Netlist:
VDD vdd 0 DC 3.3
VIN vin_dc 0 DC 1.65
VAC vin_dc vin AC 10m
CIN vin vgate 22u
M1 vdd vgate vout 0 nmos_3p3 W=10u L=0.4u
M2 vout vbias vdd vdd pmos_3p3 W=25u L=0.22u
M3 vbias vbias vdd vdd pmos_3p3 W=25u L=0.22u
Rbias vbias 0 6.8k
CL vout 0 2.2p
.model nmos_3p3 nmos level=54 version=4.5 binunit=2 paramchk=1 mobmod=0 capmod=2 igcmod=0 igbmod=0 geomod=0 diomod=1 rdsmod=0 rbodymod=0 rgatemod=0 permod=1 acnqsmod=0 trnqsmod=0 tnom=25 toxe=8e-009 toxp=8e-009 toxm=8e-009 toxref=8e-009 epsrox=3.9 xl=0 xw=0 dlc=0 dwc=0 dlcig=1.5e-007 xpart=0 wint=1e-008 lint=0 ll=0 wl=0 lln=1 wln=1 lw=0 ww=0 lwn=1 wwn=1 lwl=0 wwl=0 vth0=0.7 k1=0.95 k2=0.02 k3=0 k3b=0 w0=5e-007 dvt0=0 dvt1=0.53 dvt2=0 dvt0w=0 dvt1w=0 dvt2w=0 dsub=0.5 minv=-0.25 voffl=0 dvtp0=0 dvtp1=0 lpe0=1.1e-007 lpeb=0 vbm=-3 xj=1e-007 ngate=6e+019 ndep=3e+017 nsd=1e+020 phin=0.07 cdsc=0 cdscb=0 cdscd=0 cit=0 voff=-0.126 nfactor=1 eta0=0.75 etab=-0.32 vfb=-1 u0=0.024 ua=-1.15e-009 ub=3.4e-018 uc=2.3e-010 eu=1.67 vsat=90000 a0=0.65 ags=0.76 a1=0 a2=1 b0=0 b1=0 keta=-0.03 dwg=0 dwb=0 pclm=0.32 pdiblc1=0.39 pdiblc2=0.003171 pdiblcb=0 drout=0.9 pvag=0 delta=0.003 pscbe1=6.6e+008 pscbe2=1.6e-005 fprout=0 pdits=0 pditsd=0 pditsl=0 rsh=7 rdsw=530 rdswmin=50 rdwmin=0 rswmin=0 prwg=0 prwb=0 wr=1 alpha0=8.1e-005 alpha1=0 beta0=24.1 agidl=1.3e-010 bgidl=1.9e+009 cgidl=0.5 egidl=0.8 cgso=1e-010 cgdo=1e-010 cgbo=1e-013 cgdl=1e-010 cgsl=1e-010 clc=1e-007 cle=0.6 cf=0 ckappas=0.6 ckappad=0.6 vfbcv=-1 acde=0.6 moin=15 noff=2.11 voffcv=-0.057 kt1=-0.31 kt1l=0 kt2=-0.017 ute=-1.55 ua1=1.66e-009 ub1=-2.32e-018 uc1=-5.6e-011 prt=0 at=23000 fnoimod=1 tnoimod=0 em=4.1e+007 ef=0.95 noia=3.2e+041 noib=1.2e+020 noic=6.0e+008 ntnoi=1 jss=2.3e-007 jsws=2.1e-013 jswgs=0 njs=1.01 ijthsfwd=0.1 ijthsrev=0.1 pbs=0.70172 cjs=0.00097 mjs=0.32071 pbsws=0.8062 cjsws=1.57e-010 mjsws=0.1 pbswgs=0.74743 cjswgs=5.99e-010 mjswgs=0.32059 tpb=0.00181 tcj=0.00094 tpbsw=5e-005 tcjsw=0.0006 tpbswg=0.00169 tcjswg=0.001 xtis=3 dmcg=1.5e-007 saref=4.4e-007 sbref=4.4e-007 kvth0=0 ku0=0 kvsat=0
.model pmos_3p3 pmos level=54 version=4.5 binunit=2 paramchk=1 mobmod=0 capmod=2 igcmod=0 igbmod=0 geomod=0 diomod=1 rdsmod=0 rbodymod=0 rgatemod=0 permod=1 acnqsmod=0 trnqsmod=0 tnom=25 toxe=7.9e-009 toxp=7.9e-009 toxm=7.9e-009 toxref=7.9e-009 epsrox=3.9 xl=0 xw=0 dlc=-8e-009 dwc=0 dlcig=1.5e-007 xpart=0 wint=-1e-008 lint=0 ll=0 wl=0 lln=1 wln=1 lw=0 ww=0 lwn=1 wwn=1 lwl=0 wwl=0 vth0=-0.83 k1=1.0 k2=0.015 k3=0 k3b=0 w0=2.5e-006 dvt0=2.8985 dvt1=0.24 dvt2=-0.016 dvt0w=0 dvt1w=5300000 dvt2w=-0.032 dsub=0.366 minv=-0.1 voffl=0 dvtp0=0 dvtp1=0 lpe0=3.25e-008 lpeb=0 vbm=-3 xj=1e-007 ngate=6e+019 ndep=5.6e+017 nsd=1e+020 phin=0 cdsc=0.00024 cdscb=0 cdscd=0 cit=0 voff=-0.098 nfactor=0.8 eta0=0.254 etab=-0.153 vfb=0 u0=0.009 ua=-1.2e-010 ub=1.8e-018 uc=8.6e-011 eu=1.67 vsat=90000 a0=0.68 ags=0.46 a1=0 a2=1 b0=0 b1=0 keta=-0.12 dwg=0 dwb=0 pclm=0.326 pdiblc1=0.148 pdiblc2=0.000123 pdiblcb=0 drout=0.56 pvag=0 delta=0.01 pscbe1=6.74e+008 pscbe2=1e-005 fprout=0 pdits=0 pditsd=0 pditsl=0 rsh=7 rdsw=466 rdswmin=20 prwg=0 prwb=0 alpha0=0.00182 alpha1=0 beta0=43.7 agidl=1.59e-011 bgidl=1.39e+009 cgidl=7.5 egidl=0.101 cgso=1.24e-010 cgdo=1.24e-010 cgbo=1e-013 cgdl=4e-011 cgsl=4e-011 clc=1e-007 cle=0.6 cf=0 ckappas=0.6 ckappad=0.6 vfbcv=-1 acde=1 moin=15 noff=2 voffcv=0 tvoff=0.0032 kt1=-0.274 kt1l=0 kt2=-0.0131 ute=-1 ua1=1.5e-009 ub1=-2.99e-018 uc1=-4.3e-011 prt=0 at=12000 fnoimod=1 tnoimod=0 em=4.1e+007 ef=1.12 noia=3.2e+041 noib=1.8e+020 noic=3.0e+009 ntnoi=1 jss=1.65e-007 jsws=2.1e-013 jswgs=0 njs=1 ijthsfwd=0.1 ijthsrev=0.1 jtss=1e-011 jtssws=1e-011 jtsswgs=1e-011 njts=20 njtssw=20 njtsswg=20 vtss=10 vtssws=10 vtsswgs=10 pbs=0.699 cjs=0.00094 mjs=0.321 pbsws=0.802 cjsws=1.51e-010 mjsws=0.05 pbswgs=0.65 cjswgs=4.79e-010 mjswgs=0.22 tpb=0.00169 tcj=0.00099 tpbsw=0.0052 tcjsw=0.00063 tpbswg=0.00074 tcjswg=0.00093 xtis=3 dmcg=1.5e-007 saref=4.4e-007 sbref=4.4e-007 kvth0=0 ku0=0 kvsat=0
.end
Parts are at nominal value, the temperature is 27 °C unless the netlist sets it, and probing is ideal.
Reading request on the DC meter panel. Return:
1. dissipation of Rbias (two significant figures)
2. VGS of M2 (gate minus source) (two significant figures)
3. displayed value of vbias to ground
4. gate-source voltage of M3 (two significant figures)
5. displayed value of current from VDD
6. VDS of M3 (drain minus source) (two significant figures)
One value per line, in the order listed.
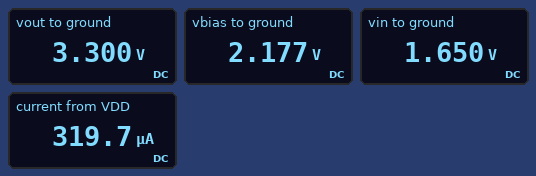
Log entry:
700 µW
-1.1 V
2.177 V
-1.1 V
319.7 µA
-1.1 V
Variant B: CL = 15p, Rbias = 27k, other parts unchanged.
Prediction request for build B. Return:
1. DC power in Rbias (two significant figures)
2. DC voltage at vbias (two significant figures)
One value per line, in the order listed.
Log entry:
210 µW
2.4 V
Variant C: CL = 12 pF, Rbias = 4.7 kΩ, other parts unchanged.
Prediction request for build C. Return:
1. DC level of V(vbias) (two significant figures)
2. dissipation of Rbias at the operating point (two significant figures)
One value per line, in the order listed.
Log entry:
2.1 V
930 µW
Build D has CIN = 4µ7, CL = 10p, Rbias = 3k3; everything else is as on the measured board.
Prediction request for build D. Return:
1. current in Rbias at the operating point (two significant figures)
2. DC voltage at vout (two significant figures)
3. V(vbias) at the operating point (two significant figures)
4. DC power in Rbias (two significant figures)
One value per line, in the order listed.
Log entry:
610 µA
3.3 V
2.0 V
1.2 mW
